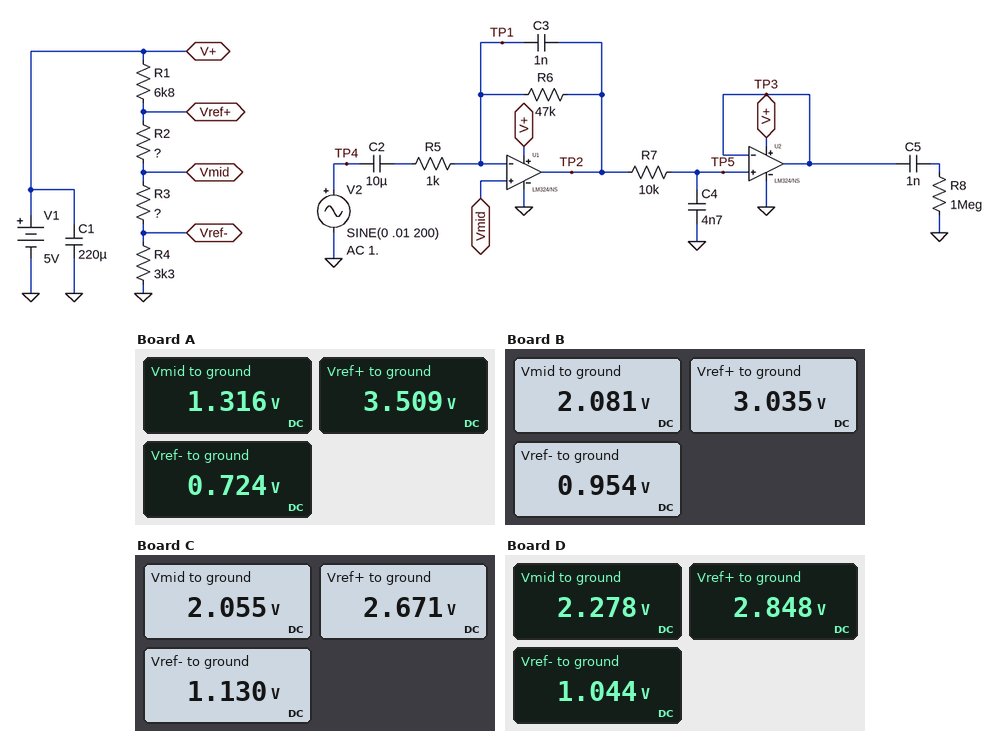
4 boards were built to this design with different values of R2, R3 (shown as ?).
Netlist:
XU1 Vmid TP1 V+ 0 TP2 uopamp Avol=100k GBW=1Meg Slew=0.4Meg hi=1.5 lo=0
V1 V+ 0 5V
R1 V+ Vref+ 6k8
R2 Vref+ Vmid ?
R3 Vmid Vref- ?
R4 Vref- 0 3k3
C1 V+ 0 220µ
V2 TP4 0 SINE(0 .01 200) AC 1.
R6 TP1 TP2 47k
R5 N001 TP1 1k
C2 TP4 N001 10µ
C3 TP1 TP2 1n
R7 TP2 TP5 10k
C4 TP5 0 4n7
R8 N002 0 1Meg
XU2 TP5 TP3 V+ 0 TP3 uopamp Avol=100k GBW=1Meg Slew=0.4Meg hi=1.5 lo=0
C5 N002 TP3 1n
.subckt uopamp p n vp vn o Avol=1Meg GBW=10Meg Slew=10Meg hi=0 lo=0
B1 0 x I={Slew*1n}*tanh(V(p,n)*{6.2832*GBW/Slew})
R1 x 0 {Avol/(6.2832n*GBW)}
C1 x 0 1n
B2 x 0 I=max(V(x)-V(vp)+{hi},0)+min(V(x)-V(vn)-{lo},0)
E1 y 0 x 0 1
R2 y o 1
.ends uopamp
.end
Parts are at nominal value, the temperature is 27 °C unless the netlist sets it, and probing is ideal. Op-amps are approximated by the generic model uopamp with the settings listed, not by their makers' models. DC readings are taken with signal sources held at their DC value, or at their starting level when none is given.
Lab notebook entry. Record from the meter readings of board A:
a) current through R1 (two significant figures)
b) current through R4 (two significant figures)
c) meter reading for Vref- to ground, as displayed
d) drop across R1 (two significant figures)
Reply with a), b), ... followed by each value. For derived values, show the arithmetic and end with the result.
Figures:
a) (5 V - 3.509 V) / 6.8 kΩ = 220 µA
b) (724 mV) / 3.3 kΩ = 220 µA
c) 0.724 V
d) 5 V - 3.509 V = 1.5 V
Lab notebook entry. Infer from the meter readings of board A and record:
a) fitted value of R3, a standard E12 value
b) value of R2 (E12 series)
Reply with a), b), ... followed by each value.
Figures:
a) 2.7 kΩ
b) 10 kΩ
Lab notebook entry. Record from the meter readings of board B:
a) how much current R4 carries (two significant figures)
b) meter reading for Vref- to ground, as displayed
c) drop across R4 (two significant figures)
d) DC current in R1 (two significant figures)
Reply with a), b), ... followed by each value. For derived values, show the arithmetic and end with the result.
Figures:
a) (954 mV) / 3.3 kΩ = 290 µA
b) 0.954 V
c) 954 mV = 950 mV
d) (5 V - 3.035 V) / 6.8 kΩ = 290 µA
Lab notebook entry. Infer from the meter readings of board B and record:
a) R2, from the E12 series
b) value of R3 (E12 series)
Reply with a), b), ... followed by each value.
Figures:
a) 3.3 kΩ
b) 3.9 kΩ
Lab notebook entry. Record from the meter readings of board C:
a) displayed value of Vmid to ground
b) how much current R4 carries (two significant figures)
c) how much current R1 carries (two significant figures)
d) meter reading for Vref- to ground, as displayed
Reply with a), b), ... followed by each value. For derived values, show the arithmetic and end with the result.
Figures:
a) 2.055 V
b) (1.13 V) / 3.3 kΩ = 340 µA
c) (5 V - 2.671 V) / 6.8 kΩ = 340 µA
d) 1.130 V
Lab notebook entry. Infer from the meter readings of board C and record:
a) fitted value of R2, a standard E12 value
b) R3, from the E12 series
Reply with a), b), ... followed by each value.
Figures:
a) 1.8 kΩ
b) 2.7 kΩ
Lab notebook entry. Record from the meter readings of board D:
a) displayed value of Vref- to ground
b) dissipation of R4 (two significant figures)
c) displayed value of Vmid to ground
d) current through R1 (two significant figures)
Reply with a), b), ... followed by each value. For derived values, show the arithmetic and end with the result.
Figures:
a) 1.044 V
b) (1.044 V)^2 / 3.3 kΩ = 330 µW
c) 2.278 V
d) (5 V - 2.848 V) / 6.8 kΩ = 320 µA
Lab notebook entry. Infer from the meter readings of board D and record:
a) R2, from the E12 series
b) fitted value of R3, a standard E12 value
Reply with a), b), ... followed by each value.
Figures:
a) 1.8 kΩ
b) 3.9 kΩ
